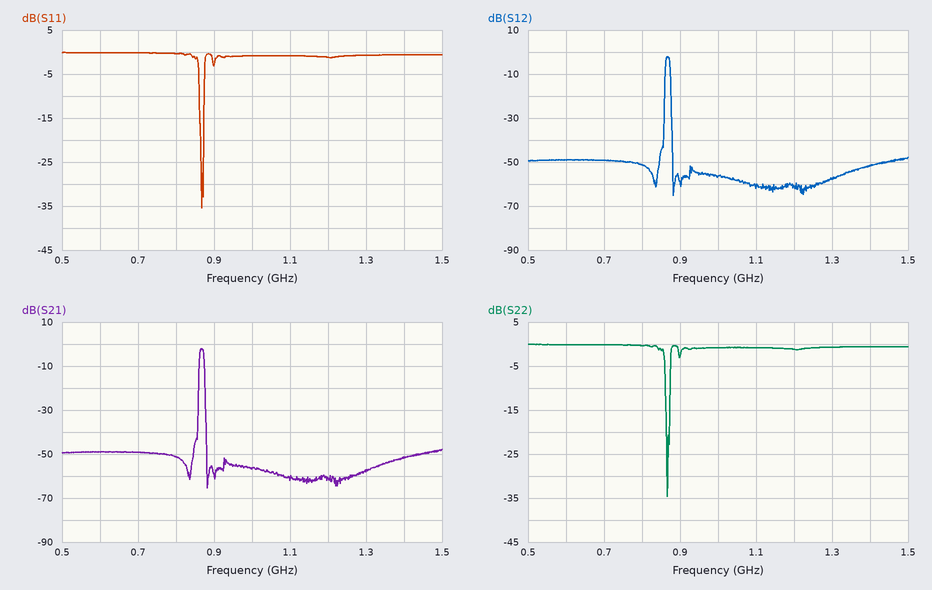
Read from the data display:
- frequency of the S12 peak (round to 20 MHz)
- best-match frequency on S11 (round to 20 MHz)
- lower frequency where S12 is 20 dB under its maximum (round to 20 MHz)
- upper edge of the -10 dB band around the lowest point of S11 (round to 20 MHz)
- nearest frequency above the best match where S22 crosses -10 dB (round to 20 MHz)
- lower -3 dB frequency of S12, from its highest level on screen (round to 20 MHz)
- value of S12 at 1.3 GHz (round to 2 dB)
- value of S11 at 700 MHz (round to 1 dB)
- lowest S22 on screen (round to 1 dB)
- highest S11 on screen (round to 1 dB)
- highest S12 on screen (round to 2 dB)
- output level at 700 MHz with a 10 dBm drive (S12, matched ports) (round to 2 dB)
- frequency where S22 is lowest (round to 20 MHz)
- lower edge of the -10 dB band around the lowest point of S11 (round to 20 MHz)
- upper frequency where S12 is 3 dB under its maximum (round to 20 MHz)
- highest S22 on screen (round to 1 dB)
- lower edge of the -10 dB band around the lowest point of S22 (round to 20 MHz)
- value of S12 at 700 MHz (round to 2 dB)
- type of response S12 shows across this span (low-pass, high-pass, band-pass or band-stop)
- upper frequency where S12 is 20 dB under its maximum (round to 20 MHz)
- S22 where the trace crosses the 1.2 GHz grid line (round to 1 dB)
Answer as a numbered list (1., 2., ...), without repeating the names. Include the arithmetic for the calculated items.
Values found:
1. 860 MHz
2. 860 MHz
3. 860 MHz
4. 880 MHz
5. 880 MHz
6. 860 MHz
7. -58 dB
8. 0 dB
9. -35 dB
10. 0 dB
11. -2 dB
12. 10 dBm + (-50 dB) = -40 dBm
13. 860 MHz
14. 860 MHz
15. 880 MHz
16. 0 dB
17. 860 MHz
18. -50 dB
19. band-pass
20. 880 MHz
21. -1 dB
